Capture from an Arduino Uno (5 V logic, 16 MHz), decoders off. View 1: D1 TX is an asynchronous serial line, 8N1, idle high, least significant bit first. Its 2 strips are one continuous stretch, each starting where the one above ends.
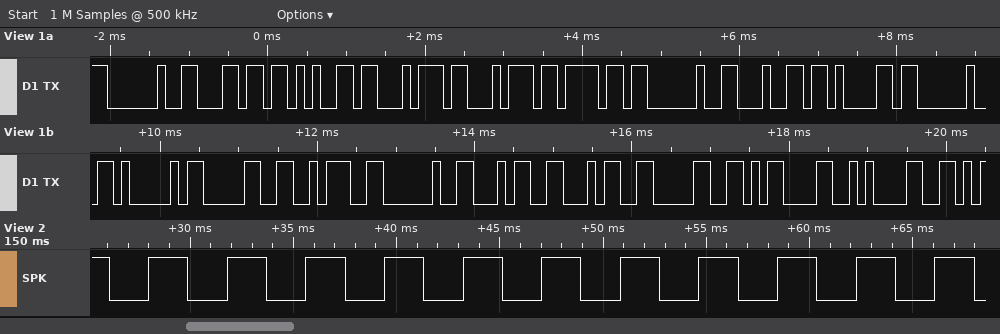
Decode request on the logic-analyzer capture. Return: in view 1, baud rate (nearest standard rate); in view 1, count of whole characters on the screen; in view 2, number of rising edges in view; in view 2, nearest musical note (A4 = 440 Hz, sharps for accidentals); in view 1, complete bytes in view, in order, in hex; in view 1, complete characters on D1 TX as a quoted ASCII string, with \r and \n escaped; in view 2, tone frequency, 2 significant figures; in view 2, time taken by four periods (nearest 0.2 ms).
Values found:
9600 baud
19
11
C4
20 6C 65 74 74 6F 20 64 61 20 41 30 3A 20 34 34 30 0D 0A
" letto da A0: 440\r\n"
260 Hz
15.2 ms
